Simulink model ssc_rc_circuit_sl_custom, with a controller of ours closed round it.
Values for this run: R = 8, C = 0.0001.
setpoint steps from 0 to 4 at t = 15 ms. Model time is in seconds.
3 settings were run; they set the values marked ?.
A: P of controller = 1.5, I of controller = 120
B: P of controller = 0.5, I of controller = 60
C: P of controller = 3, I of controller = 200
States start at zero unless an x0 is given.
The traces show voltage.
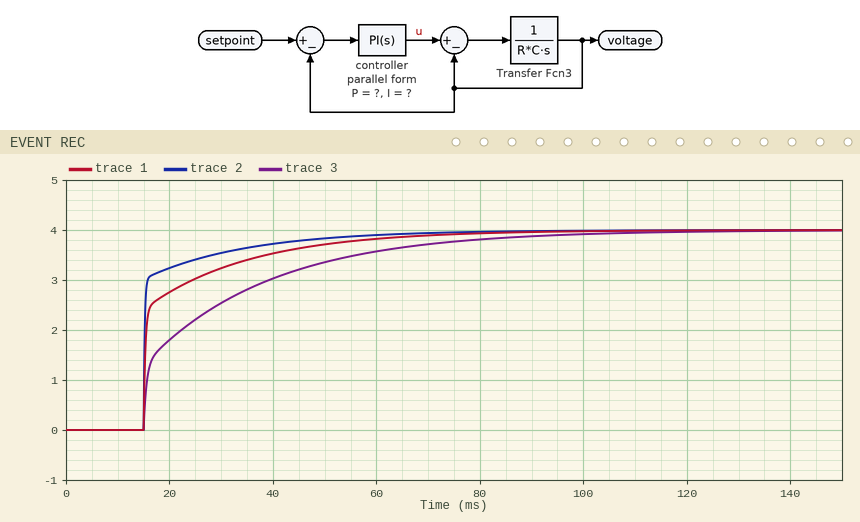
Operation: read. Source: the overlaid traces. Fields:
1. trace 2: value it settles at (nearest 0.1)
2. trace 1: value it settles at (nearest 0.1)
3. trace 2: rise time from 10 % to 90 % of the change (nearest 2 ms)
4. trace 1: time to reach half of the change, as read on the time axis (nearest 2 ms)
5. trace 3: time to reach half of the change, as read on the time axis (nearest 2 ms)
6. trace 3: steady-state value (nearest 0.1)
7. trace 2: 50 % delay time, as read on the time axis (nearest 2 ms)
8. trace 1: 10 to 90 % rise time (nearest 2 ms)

4.0
4.0
18 ms
16 ms
22 ms
4.0
16 ms
28 ms
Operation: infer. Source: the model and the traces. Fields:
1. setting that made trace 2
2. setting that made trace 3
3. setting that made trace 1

C
B
A
